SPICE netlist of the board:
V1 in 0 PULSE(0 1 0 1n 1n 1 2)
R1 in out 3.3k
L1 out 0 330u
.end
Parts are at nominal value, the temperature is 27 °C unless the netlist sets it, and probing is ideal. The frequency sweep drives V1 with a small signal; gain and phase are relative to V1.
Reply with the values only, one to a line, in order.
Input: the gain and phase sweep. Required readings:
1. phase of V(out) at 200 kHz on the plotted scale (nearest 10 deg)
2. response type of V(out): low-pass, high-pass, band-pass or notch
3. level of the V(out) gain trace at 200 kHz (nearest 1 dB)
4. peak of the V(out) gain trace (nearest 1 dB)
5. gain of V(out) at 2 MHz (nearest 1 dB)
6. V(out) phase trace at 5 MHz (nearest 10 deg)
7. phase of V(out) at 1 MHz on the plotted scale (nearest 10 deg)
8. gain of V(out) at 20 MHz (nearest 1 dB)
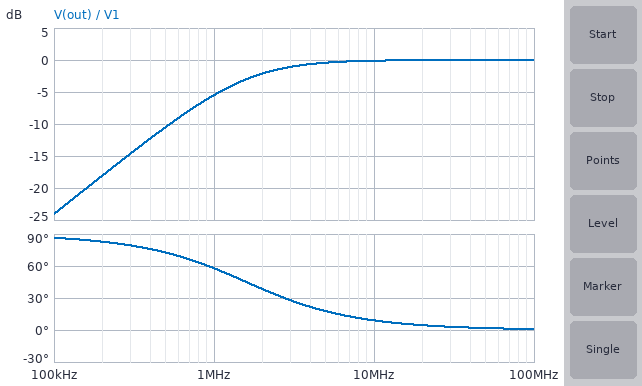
80 deg
high-pass
-18 dB
0 dB
-2 dB
20 deg
60 deg
0 dB
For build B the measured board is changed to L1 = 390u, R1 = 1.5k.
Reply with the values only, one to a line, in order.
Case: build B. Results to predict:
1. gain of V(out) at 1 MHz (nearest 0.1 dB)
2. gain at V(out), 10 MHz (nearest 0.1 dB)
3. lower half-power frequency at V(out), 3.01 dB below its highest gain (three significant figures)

-1.4 dB
0 dB
612 kHz
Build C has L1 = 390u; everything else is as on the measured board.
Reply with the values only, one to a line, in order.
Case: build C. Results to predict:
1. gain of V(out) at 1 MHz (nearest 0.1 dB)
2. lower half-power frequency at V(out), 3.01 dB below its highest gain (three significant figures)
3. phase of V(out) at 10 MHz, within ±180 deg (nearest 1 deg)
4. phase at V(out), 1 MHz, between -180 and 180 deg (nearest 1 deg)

-4.5 dB
1.35 MHz
8 deg
53 deg
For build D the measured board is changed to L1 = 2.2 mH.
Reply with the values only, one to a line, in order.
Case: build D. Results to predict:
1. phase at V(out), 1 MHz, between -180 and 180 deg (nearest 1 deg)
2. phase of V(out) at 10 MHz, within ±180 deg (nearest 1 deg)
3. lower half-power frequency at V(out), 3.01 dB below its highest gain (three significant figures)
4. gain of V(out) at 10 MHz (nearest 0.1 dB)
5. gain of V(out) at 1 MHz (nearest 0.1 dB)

13 deg
1 deg
239 kHz
0 dB
-0.2 dB
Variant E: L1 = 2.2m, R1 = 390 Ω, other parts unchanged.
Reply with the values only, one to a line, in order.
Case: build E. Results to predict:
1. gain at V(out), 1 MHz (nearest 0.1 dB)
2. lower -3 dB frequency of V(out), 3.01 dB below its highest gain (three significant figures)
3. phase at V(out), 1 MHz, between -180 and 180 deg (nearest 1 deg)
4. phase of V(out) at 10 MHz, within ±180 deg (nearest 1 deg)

0 dB
28.2 kHz
2 deg
0 deg
